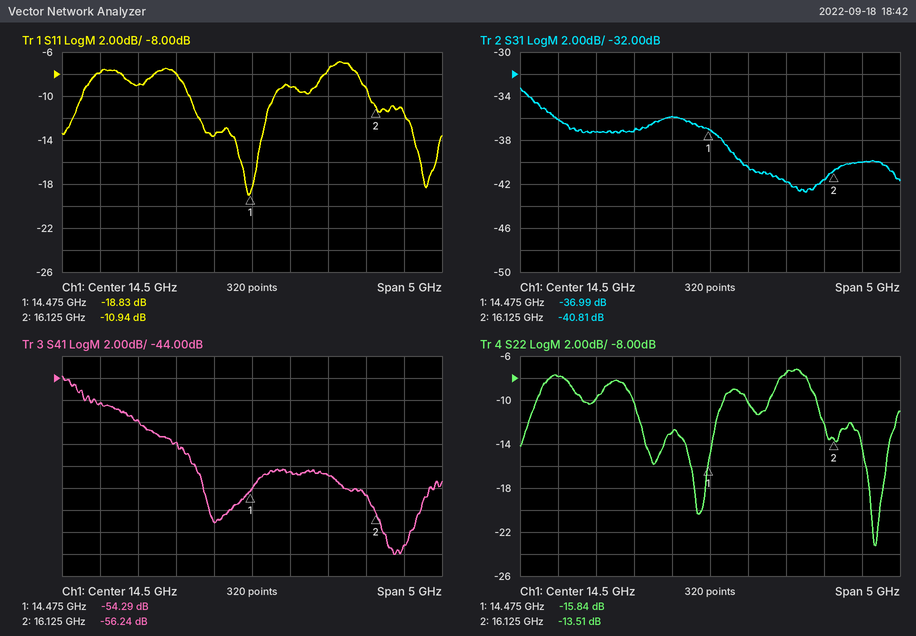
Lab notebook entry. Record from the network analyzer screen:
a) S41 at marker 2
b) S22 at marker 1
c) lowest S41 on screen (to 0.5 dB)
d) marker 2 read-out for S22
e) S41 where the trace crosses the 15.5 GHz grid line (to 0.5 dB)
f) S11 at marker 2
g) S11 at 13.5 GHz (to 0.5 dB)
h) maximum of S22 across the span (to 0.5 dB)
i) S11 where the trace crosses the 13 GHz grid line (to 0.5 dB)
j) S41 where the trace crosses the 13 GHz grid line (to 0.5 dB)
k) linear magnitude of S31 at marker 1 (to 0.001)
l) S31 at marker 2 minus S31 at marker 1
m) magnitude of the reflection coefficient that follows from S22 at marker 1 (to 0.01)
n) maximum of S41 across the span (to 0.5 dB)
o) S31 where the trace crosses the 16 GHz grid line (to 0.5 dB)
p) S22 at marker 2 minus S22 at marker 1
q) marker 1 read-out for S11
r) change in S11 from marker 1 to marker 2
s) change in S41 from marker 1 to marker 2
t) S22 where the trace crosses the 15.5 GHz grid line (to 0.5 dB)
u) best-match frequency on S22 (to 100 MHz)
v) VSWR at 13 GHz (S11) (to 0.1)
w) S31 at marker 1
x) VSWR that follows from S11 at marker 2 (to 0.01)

-56.24 dB
-15.84 dB
-60.0 dB
-13.51 dB
-53.0 dB
-10.94 dB
-8.0 dB
-7.0 dB
-9.0 dB
-48.0 dB
0.014
-3.82 dB
0.16
-44.0 dB
-41.5 dB
2.33 dB
-18.83 dB
7.89 dB
-1.95 dB
-7.5 dB
16.7 GHz
2.1
-36.99 dB
1.79
